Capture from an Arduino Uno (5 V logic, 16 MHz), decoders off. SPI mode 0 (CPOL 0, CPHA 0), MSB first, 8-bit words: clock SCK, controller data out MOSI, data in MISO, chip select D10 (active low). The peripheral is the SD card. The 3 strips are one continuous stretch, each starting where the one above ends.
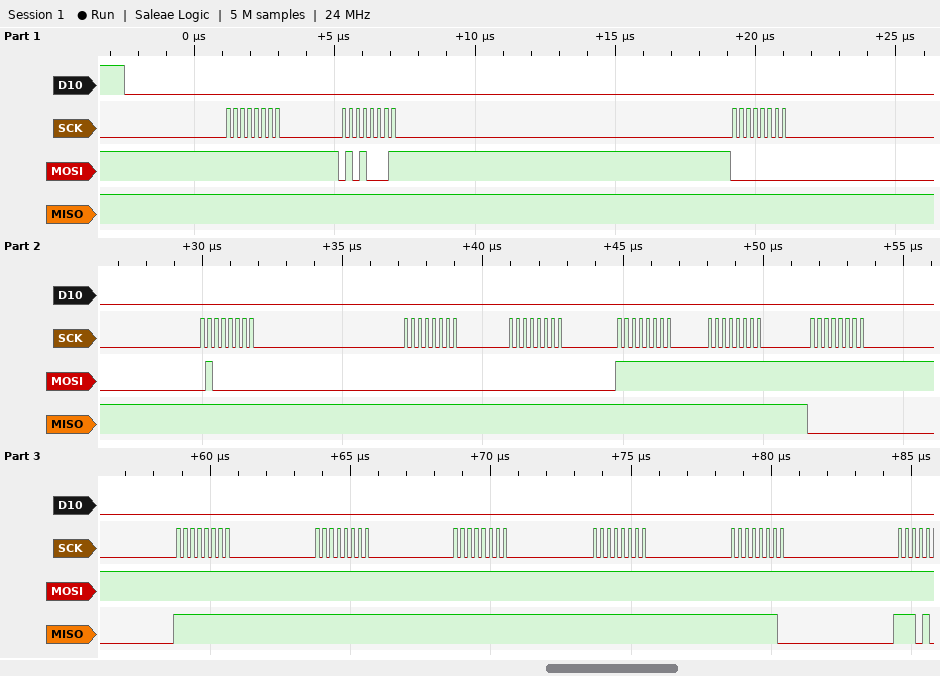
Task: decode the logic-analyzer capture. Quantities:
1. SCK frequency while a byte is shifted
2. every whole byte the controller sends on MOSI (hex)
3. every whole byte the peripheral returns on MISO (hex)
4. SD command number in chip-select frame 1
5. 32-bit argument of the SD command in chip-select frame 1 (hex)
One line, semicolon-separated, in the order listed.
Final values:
4 MHz; FF 51 00 40 00 00 FF FF FF FF FF FF FF FF; FF FF FF FF FF FF FF FF 00 FF FF FF FF FE; CMD17; 0x00400000
